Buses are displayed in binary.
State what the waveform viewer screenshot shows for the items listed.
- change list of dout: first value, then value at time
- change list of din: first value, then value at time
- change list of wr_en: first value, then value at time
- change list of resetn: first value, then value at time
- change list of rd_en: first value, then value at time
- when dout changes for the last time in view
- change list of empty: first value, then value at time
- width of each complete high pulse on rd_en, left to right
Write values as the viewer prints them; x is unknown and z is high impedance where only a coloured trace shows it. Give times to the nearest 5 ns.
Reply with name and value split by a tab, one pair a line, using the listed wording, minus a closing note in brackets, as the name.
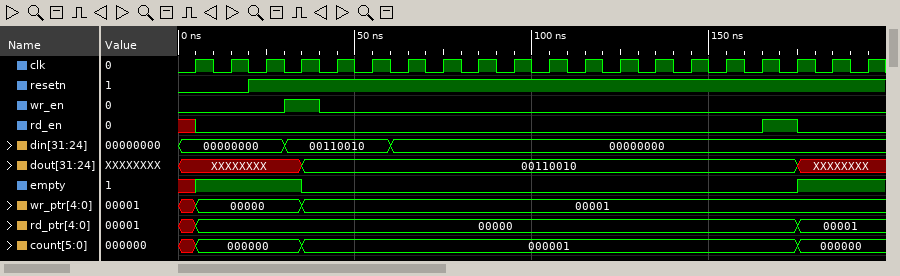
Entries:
change list of dout: first value, then value at time	XXXXXXXX, 00110010 at 35 ns, XXXXXXXX at 175 ns
change list of din: first value, then value at time	00000000, 00110010 at 30 ns, 00000000 at 60 ns
change list of wr_en: first value, then value at time	0, 1 at 30 ns, 0 at 40 ns
change list of resetn: first value, then value at time	0, 1 at 20 ns
change list of rd_en: first value, then value at time	x, 0 at 5 ns, 1 at 165 ns, 0 at 175 ns
when dout changes for the last time in view	175 ns
change list of empty: first value, then value at time	x, 1 at 5 ns, 0 at 35 ns, 1 at 175 ns
width of each complete high pulse on rd_en, left to right	10 ns
